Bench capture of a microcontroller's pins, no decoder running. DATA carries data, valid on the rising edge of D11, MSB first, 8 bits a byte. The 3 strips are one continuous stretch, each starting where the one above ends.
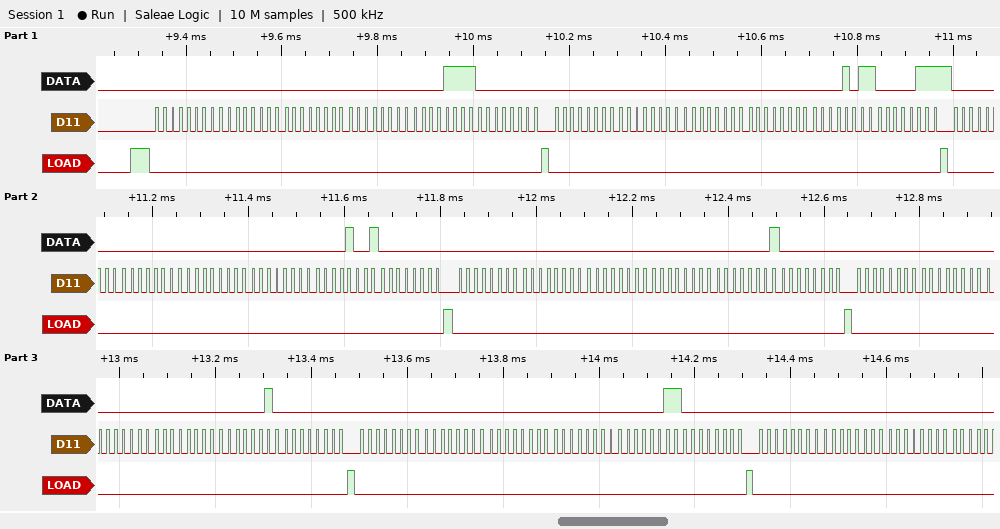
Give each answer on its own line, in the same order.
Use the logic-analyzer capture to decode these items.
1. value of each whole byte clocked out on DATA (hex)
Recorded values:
00 00 00 00 0F 00 00 00 00 00 0B 07 00 00 00 00 09 00 00 00 00 00 01 00 00 00 00 00 02 00 00 00 00 00 03 00 00 00 00
